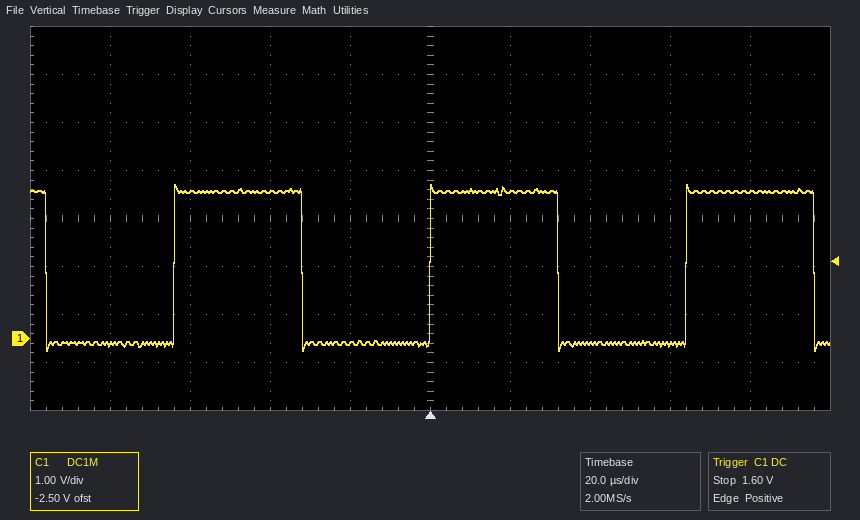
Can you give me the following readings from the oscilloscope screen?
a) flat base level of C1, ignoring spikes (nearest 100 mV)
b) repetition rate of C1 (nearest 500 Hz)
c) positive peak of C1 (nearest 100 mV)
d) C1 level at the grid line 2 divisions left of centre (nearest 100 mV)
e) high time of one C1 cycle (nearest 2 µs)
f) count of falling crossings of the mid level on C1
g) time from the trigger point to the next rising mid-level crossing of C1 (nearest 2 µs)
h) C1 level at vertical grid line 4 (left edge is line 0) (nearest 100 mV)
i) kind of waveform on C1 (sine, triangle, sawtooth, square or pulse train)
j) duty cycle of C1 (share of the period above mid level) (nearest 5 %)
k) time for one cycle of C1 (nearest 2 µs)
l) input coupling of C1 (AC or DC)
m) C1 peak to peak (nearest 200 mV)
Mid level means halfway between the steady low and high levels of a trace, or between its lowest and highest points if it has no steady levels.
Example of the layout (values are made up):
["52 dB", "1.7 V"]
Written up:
["-100 mV", "15.5 kHz", "3.2 V", "3.1 V", "32 µs", "4", "64 µs", "-100 mV", "square", "50 %", "64 µs", "DC", "3.4 V"]
